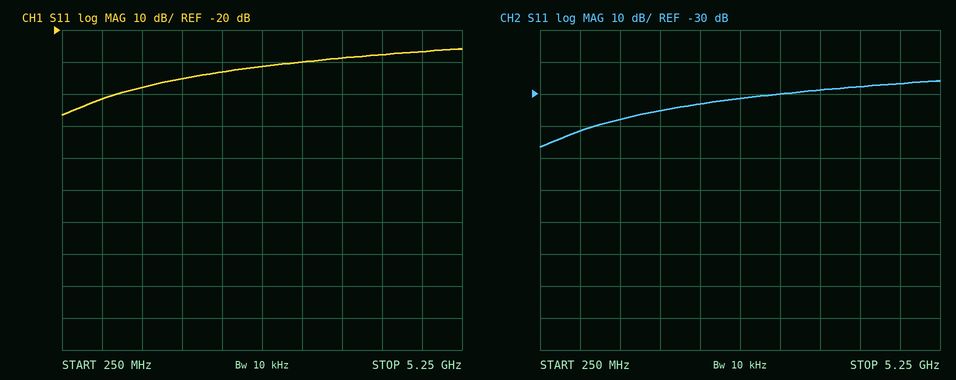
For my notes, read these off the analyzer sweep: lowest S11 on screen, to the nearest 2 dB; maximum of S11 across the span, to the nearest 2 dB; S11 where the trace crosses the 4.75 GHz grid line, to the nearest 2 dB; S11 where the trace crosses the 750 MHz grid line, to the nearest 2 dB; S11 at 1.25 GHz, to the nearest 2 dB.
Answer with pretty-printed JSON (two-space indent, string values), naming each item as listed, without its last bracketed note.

{
  "lowest S11 on screen, to the nearest 2 dB": "-46 dB",
  "maximum of S11 across the span, to the nearest 2 dB": "-26 dB",
  "S11 where the trace crosses the 4.75 GHz grid line, to the nearest 2 dB": "-26 dB",
  "S11 where the trace crosses the 750 MHz grid line, to the nearest 2 dB": "-42 dB",
  "S11 at 1.25 GHz, to the nearest 2 dB": "-38 dB"
}
